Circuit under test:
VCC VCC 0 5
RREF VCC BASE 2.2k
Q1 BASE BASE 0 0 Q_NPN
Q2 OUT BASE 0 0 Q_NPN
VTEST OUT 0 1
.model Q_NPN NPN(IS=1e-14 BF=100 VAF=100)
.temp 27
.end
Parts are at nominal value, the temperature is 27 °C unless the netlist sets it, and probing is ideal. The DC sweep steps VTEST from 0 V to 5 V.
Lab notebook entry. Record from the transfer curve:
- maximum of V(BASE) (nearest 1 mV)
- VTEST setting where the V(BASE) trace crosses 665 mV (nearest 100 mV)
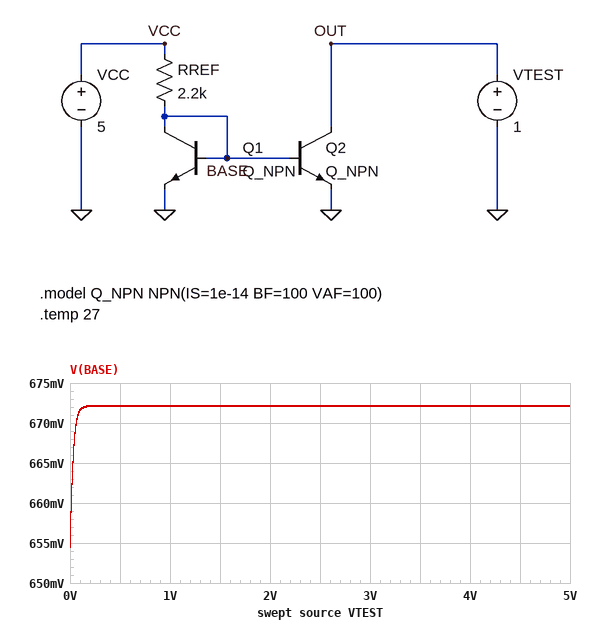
672 mV
0 V
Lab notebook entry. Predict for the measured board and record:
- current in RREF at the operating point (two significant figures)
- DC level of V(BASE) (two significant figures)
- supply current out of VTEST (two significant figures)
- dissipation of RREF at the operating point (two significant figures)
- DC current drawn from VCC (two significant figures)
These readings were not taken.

2.0 mA
670 mV
1.9 mA
8.5 mW
2.0 mA
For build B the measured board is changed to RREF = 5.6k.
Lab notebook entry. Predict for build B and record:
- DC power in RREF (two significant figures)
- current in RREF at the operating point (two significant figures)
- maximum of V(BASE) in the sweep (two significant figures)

3.4 mW
780 µA
650 mV
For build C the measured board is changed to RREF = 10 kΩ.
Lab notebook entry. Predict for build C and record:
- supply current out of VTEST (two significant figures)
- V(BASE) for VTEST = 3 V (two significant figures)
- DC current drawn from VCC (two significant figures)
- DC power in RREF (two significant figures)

430 µA
630 mV
440 µA
1.9 mW
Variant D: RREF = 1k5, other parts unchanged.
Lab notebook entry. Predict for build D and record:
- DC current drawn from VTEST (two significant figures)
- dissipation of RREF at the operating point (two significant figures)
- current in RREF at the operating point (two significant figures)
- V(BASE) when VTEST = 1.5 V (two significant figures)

2.8 mA
12 mW
2.9 mA
680 mV
